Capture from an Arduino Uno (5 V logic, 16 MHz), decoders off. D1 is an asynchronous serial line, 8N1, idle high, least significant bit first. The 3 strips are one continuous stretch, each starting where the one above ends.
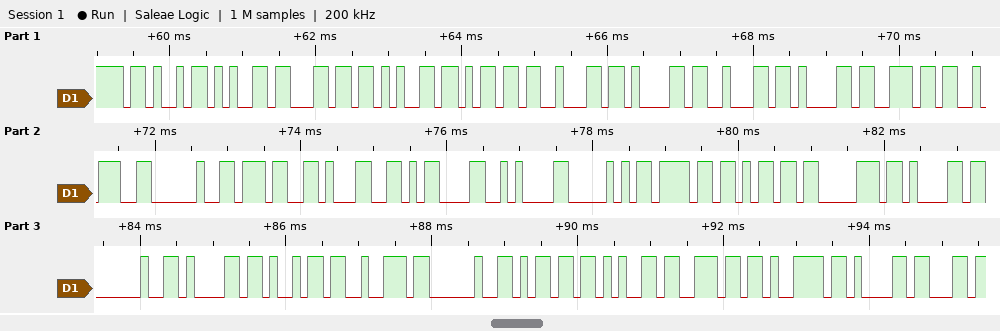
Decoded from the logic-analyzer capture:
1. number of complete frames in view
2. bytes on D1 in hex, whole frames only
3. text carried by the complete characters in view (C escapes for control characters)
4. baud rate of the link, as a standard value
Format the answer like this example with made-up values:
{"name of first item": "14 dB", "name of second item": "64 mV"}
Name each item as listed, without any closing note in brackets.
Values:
{"number of complete frames in view": "31", "bytes on D1 in hex, whole frames only": "0x4B 0x65 0x6C 0x65 0x6D 0x62 0x61 0x62 0x61 0x6E 0x3A 0x20 0x37 0x31 0x0D 0x0A 0x50 0x6F 0x6D 0x70 0x61 0x20 0x61 0x69 0x72 0x20 0x6D 0x65 0x6E 0x79 0x61", "text carried by the complete characters in view": "\"Kelembaban: 71\\r\\nPompa air menya\"", "baud rate of the link, as a standard value": "9600 baud"}
